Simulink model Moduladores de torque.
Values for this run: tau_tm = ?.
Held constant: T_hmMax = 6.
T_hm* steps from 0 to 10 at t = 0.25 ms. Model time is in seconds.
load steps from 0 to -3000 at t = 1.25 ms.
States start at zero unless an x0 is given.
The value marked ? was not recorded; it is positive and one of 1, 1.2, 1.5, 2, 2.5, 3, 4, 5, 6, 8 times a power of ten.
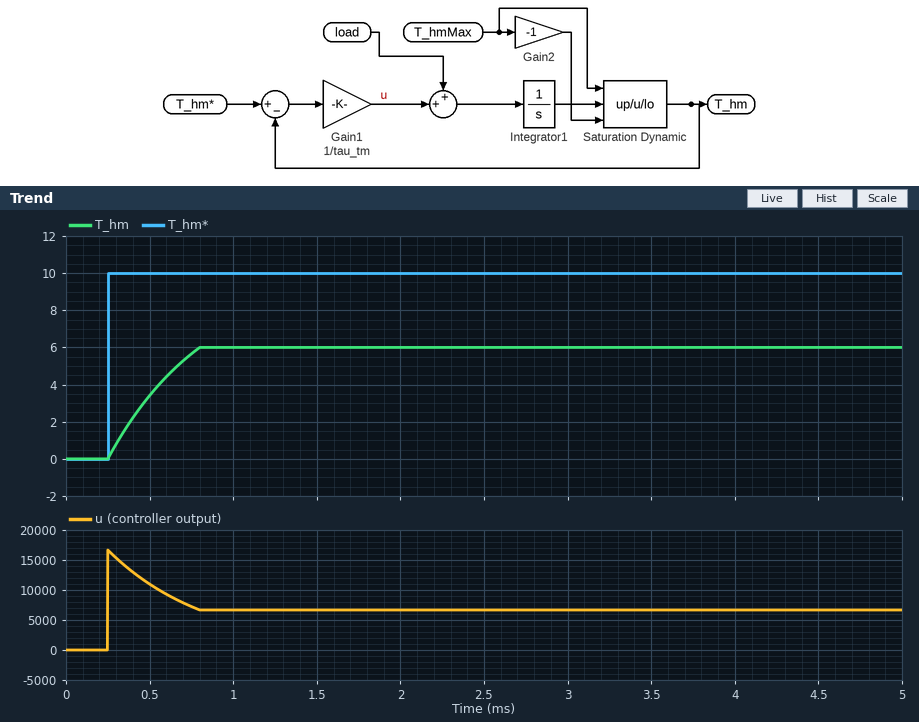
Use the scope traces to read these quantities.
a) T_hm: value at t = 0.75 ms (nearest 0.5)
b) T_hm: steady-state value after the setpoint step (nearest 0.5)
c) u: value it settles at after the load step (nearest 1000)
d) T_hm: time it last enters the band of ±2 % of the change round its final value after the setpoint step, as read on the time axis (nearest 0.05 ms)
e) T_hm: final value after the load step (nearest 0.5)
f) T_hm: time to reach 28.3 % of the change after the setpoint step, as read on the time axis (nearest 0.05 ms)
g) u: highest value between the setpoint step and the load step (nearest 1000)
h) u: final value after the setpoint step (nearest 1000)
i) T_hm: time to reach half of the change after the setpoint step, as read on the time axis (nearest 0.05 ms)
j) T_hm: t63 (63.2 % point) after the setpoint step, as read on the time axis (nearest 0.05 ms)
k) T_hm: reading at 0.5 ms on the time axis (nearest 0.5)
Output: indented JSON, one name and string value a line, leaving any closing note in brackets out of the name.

{
  "T_hm: value at t = 0.75 ms": "5.5",
  "T_hm: steady-state value after the setpoint step": "6.0",
  "u: value it settles at after the load step": "7000",
  "T_hm: time it last enters the band of ±2 % of the change round its final value after the setpoint step, as read on the time axis": "0.80 ms",
  "T_hm: final value after the load step": "6.0",
  "T_hm: time to reach 28.3 % of the change after the setpoint step, as read on the time axis": "0.35 ms",
  "u: highest value between the setpoint step and the load step": "17000",
  "u: final value after the setpoint step": "7000",
  "T_hm: time to reach half of the change after the setpoint step, as read on the time axis": "0.45 ms",
  "T_hm: t63 (63.2 % point) after the setpoint step, as read on the time axis": "0.55 ms",
  "T_hm: reading at 0.5 ms on the time axis": "3.5"
}
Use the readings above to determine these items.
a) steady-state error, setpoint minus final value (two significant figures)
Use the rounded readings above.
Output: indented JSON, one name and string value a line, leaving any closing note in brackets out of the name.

{
  "steady-state error, setpoint minus final value": "4.0"
}
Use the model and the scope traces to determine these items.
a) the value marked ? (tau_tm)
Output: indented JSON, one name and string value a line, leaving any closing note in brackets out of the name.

{
  "the value marked ?": "0.0006"
}
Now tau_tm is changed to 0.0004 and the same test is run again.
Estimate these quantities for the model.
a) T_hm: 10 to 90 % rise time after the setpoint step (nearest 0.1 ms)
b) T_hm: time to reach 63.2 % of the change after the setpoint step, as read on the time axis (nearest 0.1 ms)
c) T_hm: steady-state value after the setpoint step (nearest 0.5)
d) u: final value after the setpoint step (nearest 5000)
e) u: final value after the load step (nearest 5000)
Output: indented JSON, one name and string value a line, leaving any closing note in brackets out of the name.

{
  "T_hm: 10 to 90 % rise time after the setpoint step": "0.3 ms",
  "T_hm: time to reach 63.2 % of the change after the setpoint step, as read on the time axis": "0.4 ms",
  "T_hm: steady-state value after the setpoint step": "6.0",
  "u: final value after the setpoint step": "10000",
  "u: final value after the load step": "10000"
}
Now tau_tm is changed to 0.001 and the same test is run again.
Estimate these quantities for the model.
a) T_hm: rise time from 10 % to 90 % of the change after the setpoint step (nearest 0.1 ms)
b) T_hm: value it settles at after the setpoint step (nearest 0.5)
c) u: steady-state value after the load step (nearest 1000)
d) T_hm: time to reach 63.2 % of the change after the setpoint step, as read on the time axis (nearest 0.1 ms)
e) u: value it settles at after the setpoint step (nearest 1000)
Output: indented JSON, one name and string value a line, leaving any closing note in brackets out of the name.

{
  "T_hm: rise time from 10 % to 90 % of the change after the setpoint step": "0.7 ms",
  "T_hm: value it settles at after the setpoint step": "6.0",
  "u: steady-state value after the load step": "4000",
  "T_hm: time to reach 63.2 % of the change after the setpoint step, as read on the time axis": "0.7 ms",
  "u: value it settles at after the setpoint step": "4000"
}
